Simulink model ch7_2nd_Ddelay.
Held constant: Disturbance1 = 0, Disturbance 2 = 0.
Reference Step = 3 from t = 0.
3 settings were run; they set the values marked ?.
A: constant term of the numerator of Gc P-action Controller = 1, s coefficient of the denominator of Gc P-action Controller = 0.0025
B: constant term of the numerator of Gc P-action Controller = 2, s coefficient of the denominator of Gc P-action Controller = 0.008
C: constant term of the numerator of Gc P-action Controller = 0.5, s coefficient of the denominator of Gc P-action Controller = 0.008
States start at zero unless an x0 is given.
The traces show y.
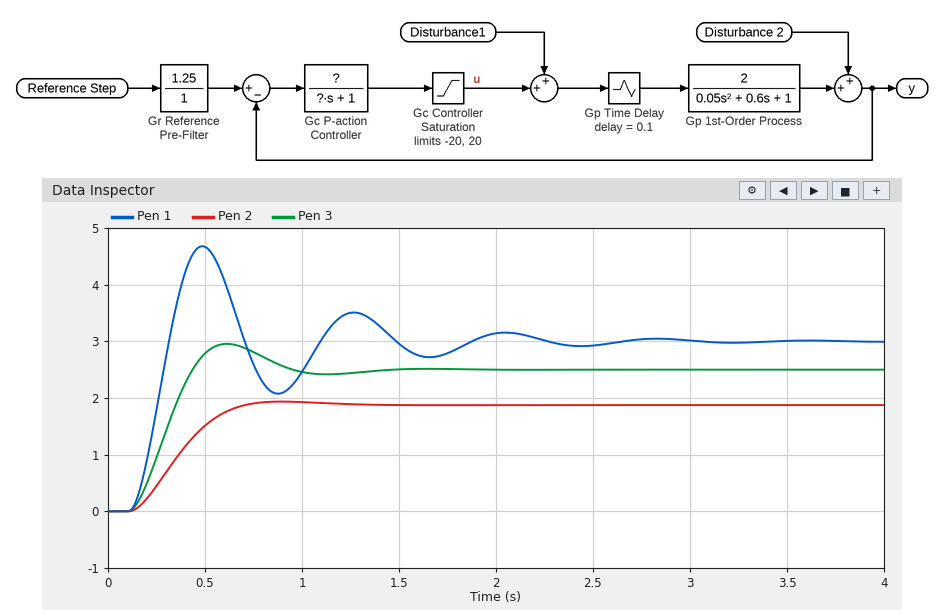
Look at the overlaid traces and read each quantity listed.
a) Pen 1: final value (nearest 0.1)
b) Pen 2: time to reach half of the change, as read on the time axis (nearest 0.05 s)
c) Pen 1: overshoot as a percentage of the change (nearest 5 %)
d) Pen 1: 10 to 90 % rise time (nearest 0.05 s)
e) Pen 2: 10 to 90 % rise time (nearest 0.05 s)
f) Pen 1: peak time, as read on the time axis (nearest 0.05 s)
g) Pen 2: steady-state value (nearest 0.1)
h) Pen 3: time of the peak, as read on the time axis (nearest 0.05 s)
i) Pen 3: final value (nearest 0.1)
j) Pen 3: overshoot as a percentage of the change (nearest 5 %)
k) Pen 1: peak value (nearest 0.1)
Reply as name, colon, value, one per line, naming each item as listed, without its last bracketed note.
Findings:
Pen 1: final value: 3.0
Pen 2: time to reach half of the change, as read on the time axis: 0.35 s
Pen 1: overshoot as a percentage of the change: 55 %
Pen 1: 10 to 90 % rise time: 0.15 s
Pen 2: 10 to 90 % rise time: 0.40 s
Pen 1: peak time, as read on the time axis: 0.50 s
Pen 2: steady-state value: 1.9
Pen 3: time of the peak, as read on the time axis: 0.60 s
Pen 3: final value: 2.5
Pen 3: overshoot as a percentage of the change: 20 %
Pen 1: peak value: 4.7
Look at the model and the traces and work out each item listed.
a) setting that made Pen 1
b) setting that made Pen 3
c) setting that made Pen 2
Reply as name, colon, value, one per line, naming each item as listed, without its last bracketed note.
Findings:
setting that made Pen 1: B
setting that made Pen 3: A
setting that made Pen 2: C
